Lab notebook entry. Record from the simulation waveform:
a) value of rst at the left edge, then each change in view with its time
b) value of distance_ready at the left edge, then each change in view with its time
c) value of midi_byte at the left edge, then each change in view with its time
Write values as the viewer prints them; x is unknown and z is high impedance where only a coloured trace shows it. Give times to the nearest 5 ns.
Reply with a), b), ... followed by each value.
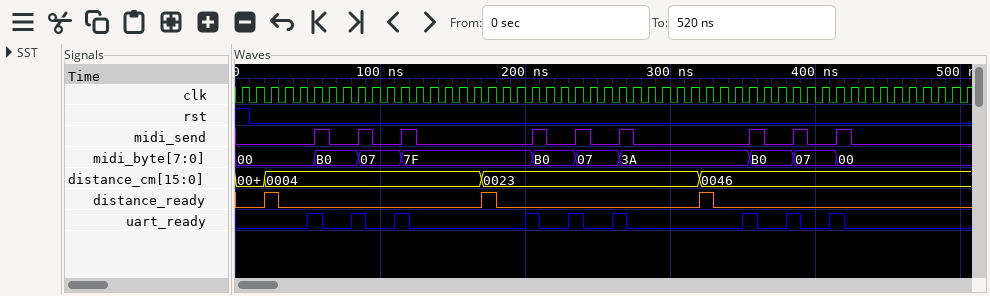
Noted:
a) 1, 0 at 10 ns
b) 0, 1 at 20 ns, 0 at 30 ns, 1 at 170 ns, 0 at 180 ns, 1 at 320 ns, 0 at 330 ns
c) 00, B0 at 55 ns, 07 at 85 ns, 7F at 115 ns, B0 at 205 ns, 07 at 235 ns, 3A at 265 ns, B0 at 355 ns, 07 at 385 ns, 00 at 415 ns
